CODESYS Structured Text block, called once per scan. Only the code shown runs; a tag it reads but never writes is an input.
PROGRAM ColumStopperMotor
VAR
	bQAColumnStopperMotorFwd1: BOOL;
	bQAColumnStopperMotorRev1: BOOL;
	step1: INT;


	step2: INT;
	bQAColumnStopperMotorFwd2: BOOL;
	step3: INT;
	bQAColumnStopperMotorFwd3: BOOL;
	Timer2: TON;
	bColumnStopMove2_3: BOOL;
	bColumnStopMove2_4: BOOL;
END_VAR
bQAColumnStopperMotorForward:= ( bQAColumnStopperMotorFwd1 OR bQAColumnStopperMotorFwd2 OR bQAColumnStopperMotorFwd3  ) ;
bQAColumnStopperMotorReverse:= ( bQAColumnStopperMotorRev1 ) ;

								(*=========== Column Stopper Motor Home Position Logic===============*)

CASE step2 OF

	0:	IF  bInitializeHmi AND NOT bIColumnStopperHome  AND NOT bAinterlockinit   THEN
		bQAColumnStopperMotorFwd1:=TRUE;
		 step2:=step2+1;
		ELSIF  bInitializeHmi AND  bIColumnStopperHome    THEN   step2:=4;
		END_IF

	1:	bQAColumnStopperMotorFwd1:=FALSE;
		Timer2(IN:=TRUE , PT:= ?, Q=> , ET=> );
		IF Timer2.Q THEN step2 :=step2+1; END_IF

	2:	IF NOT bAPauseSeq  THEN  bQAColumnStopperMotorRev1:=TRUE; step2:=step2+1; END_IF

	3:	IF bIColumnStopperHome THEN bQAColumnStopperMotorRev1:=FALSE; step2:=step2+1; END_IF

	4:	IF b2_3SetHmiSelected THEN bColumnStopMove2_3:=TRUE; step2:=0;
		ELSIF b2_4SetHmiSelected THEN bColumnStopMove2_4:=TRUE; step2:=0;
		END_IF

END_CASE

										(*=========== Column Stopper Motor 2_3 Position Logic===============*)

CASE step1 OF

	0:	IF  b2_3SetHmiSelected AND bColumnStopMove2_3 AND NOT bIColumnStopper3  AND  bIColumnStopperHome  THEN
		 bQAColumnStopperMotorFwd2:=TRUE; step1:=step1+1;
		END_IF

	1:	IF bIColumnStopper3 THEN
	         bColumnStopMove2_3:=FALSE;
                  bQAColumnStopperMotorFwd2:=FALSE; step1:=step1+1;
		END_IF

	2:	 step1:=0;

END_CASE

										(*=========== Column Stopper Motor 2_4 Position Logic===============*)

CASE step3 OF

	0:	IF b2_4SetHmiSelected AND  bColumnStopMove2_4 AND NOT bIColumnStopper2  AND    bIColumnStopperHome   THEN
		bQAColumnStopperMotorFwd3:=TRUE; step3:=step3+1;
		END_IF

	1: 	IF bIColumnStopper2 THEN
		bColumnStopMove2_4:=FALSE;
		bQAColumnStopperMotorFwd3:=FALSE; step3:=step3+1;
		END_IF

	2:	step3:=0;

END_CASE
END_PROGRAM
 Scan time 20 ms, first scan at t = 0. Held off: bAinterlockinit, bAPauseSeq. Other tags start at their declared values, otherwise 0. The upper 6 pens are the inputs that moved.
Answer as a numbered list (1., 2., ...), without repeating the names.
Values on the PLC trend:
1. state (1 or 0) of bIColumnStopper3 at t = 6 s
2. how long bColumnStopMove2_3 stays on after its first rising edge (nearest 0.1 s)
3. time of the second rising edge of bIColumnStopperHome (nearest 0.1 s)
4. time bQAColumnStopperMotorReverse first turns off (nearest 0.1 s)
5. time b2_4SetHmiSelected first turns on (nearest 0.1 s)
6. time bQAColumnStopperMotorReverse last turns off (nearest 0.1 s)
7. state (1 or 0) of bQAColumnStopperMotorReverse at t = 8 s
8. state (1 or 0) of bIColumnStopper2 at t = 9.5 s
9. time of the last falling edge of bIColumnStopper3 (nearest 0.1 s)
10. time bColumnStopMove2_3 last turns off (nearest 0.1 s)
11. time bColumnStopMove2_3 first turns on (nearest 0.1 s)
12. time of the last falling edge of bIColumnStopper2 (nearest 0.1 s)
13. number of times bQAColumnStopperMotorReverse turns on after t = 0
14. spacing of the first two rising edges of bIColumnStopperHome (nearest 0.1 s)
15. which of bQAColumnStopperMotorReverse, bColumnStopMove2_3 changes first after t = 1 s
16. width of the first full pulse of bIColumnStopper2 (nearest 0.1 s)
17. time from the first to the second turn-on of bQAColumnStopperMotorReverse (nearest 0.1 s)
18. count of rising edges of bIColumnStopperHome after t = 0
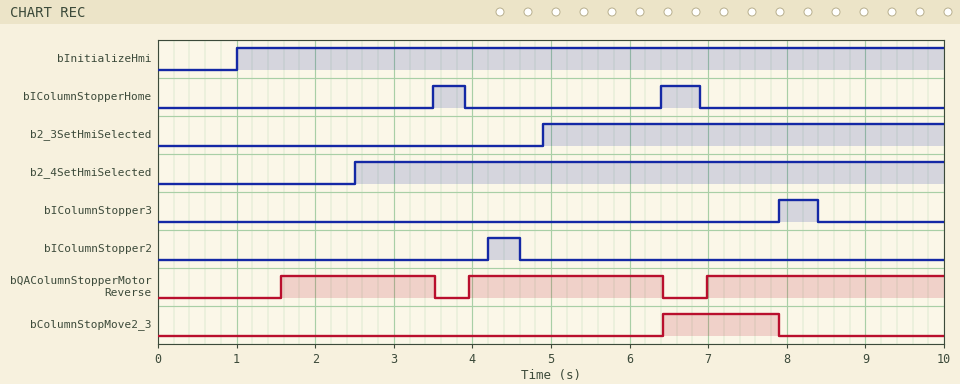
1. 0
2. 1.5 s
3. 6.4 s
4. 3.5 s
5. 2.5 s
6. 6.4 s
7. 1
8. 0
9. 8.4 s
10. 7.9 s
11. 6.4 s
12. 4.6 s
13. 3
14. 2.9 s
15. bQAColumnStopperMotorReverse
16. 0.4 s
17. 2.4 s
18. 2
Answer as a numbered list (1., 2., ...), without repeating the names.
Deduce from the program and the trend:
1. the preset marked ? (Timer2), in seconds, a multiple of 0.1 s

1. 0.5 s
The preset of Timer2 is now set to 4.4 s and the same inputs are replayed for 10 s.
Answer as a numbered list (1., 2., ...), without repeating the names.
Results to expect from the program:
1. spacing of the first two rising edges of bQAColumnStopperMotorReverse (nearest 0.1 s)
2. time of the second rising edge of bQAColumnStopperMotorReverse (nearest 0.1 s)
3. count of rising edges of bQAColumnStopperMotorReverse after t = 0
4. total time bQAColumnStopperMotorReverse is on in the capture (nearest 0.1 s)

1. 1.5 s
2. 7.0 s
3. 2
4. 4.0 s
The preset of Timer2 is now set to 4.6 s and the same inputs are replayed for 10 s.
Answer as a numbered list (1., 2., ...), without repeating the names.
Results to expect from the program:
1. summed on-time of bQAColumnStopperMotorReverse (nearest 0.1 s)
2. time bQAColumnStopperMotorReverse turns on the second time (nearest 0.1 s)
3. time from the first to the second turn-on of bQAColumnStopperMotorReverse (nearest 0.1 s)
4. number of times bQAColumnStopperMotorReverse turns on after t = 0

1. 3.8 s
2. 7.0 s
3. 1.3 s
4. 2
